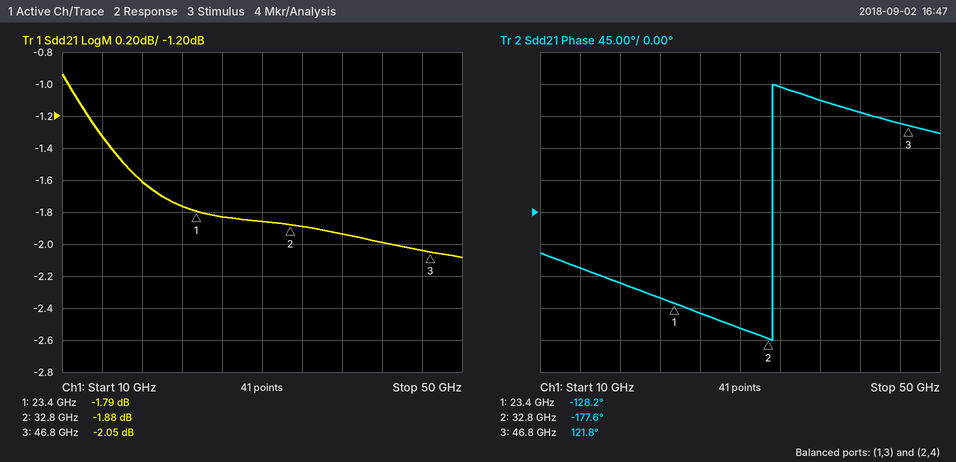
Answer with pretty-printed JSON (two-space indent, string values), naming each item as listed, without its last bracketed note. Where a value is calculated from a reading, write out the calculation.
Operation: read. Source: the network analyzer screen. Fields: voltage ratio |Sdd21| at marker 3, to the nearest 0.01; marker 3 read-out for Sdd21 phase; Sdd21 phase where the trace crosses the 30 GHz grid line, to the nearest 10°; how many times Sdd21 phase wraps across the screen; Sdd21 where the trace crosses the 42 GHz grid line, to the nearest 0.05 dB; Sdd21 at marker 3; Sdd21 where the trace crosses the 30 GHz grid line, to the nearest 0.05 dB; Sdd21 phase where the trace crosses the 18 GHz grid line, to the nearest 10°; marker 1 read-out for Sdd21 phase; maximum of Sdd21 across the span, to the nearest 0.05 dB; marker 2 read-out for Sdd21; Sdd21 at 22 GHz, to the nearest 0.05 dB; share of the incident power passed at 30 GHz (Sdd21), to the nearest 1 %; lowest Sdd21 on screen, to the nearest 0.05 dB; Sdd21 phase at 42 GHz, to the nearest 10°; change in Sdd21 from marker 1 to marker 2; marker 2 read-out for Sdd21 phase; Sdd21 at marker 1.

{
  "voltage ratio |Sdd21| at marker 3, to the nearest 0.01": "10^(-2.05/20) ≈ 0.79",
  "marker 3 read-out for Sdd21 phase": "121.8°",
  "Sdd21 phase where the trace crosses the 30 GHz grid line, to the nearest 10°": "-160°",
  "how many times Sdd21 phase wraps across the screen": "1",
  "Sdd21 where the trace crosses the 42 GHz grid line, to the nearest 0.05 dB": "-2.00 dB",
  "Sdd21 at marker 3": "-2.05 dB",
  "Sdd21 where the trace crosses the 30 GHz grid line, to the nearest 0.05 dB": "-1.85 dB",
  "Sdd21 phase where the trace crosses the 18 GHz grid line, to the nearest 10°": "-100°",
  "marker 1 read-out for Sdd21 phase": "-128.2°",
  "maximum of Sdd21 across the span, to the nearest 0.05 dB": "-0.95 dB",
  "marker 2 read-out for Sdd21": "-1.88 dB",
  "Sdd21 at 22 GHz, to the nearest 0.05 dB": "-1.75 dB",
  "share of the incident power passed at 30 GHz (Sdd21), to the nearest 1 %": "10^(-1.85/10) ≈ 65 %",
  "lowest Sdd21 on screen, to the nearest 0.05 dB": "-2.10 dB",
  "Sdd21 phase at 42 GHz, to the nearest 10°": "140°",
  "change in Sdd21 from marker 1 to marker 2": "-1.88 − (-1.79) = -0.09 dB",
  "marker 2 read-out for Sdd21 phase": "-177.6°",
  "Sdd21 at marker 1": "-1.79 dB"
}
